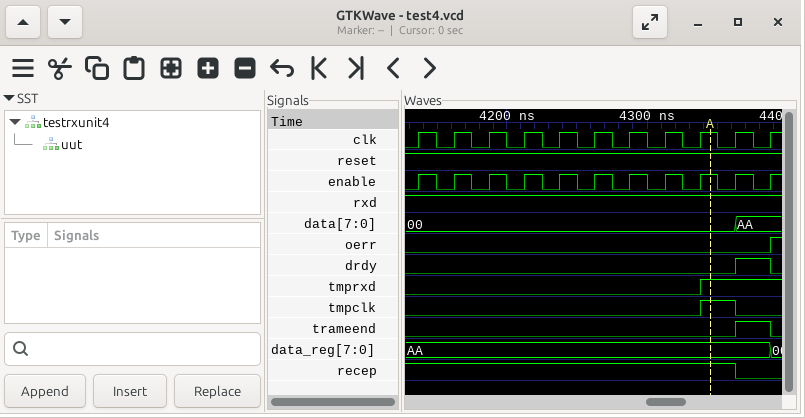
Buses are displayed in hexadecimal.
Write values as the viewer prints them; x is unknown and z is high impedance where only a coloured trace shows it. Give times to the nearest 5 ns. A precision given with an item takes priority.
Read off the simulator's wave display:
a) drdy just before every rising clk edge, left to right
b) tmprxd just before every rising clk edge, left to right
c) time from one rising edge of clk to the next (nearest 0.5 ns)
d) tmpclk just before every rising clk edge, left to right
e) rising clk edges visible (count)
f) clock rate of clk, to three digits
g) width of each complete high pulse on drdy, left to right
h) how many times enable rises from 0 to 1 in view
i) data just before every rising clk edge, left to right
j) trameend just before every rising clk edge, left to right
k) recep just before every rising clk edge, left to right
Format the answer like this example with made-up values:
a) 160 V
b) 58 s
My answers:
a) 0 0 0 0 0 0 0 0 0 0 1
b) 0 0 0 0 0 0 0 0 0 1 1
c) 25 ns
d) 0 0 0 0 0 0 0 0 0 1 0
e) 11
f) 40.0 MHz
g) 25 ns
h) 11
i) 00, 00, 00, 00, 00, 00, 00, 00, 00, 00, AA
j) 0 0 0 0 0 0 0 0 0 0 1
k) 1 1 1 1 1 1 1 1 1 1 0
